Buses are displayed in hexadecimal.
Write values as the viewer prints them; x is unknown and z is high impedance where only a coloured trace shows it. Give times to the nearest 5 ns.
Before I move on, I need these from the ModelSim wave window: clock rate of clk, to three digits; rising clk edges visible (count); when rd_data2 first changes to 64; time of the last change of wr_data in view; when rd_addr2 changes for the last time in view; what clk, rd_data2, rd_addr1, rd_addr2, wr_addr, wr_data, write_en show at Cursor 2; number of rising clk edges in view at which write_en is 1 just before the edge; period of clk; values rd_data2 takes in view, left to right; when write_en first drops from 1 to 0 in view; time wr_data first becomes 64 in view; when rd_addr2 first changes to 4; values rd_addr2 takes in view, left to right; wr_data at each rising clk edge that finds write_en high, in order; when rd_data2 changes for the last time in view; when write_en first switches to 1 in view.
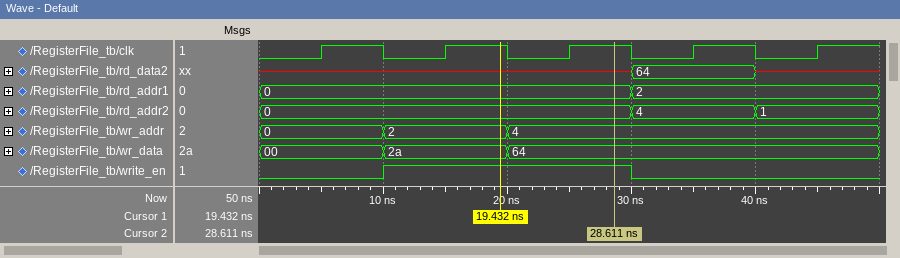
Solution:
100 MHz
5
30 ns
20 ns
40 ns
clk=1, rd_data2=x, rd_addr1=0, rd_addr2=0, wr_addr=4, wr_data=64, write_en=1
2
10 ns
x, 64, x
30 ns
20 ns
30 ns
0, 4, 1
2a, 64
40 ns
10 ns
